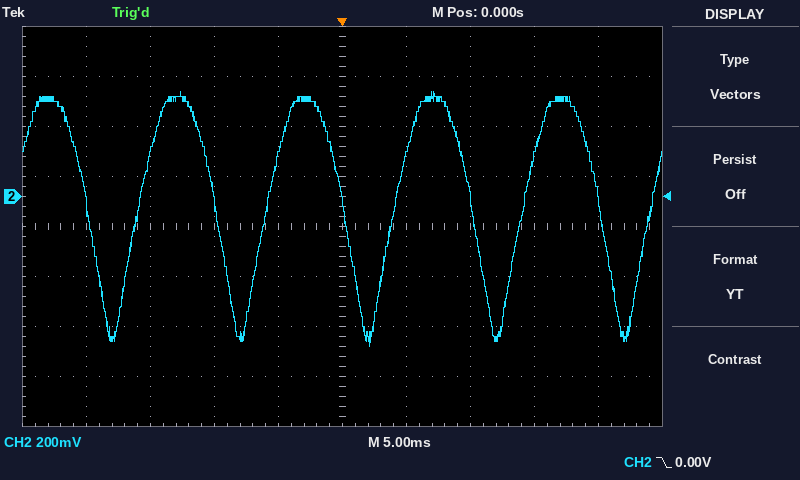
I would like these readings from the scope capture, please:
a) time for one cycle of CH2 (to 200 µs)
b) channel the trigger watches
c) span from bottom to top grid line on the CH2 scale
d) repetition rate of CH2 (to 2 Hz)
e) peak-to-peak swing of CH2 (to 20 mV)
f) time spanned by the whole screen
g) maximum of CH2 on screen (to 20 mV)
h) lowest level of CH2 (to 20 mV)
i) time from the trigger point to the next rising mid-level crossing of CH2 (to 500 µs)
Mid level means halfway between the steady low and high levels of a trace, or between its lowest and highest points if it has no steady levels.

10.0 ms
CH2
1.6 V
100 Hz
1.02 V
50 ms
420 mV
-600 mV
4.0 ms
